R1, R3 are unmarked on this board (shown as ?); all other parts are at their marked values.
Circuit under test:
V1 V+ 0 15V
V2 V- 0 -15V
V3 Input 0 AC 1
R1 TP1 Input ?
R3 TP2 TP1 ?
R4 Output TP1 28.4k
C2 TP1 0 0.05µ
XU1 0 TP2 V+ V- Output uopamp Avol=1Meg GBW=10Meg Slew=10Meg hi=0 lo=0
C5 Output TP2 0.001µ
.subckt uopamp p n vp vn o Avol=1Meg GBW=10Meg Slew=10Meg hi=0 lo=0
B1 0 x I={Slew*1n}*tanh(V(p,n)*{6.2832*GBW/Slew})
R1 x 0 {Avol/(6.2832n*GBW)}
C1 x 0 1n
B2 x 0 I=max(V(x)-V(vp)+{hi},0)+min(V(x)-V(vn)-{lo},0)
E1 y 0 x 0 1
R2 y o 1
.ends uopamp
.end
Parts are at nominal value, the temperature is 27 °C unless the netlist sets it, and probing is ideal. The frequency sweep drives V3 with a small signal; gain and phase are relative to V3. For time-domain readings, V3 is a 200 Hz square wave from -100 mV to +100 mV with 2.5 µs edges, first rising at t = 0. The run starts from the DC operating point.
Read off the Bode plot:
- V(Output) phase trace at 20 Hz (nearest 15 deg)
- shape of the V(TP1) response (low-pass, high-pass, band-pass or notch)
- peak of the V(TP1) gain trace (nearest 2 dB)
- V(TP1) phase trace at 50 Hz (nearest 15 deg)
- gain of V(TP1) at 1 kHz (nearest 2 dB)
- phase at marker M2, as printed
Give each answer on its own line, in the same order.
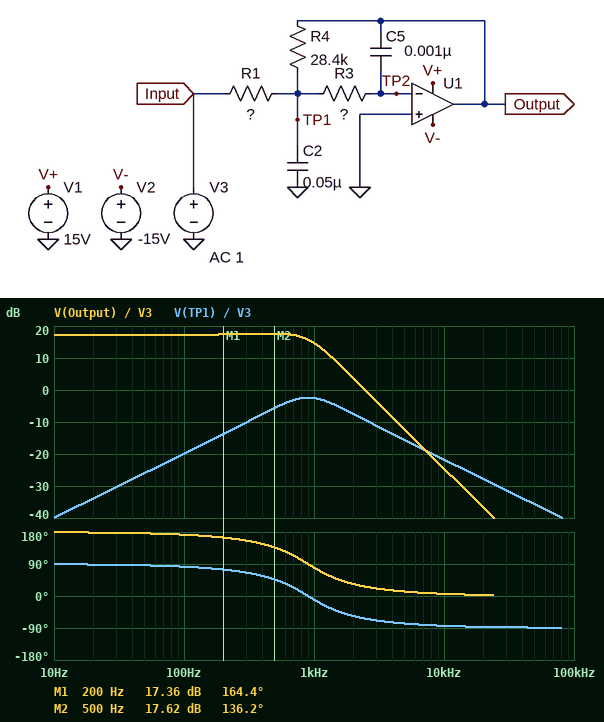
180 deg
band-pass
-2 dB
90 deg
-2 dB
136.2 deg
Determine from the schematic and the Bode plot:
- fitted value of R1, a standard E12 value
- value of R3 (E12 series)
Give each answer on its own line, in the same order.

3.9 kΩ
22 kΩ
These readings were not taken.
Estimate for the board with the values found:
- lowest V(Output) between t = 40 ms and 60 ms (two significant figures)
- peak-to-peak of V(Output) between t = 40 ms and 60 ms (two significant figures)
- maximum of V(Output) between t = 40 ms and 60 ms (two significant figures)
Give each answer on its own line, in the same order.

-870 mV
1.7 V
870 mV
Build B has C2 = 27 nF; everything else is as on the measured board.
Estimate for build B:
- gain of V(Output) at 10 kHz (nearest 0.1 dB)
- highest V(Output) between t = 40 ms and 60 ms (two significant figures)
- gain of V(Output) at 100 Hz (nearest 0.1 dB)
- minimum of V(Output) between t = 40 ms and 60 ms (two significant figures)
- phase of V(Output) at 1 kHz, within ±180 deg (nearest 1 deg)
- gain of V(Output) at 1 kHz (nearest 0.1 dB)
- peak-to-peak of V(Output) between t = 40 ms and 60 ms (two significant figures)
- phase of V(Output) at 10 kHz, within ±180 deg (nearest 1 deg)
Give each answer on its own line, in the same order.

-19.3 dB
750 mV
17.2 dB
-750 mV
104 deg
14.5 dB
1.5 V
11 deg
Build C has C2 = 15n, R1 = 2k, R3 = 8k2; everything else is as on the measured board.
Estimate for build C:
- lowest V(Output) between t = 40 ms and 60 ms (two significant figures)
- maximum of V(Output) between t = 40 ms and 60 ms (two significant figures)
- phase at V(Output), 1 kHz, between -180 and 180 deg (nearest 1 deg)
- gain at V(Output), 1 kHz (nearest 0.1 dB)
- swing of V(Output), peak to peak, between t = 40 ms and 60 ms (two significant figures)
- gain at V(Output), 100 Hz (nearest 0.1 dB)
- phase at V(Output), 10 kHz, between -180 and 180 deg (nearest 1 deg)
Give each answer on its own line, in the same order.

-1.4 V
1.4 V
132 deg
20.8 dB
2.8 V
23.0 dB
37 deg
